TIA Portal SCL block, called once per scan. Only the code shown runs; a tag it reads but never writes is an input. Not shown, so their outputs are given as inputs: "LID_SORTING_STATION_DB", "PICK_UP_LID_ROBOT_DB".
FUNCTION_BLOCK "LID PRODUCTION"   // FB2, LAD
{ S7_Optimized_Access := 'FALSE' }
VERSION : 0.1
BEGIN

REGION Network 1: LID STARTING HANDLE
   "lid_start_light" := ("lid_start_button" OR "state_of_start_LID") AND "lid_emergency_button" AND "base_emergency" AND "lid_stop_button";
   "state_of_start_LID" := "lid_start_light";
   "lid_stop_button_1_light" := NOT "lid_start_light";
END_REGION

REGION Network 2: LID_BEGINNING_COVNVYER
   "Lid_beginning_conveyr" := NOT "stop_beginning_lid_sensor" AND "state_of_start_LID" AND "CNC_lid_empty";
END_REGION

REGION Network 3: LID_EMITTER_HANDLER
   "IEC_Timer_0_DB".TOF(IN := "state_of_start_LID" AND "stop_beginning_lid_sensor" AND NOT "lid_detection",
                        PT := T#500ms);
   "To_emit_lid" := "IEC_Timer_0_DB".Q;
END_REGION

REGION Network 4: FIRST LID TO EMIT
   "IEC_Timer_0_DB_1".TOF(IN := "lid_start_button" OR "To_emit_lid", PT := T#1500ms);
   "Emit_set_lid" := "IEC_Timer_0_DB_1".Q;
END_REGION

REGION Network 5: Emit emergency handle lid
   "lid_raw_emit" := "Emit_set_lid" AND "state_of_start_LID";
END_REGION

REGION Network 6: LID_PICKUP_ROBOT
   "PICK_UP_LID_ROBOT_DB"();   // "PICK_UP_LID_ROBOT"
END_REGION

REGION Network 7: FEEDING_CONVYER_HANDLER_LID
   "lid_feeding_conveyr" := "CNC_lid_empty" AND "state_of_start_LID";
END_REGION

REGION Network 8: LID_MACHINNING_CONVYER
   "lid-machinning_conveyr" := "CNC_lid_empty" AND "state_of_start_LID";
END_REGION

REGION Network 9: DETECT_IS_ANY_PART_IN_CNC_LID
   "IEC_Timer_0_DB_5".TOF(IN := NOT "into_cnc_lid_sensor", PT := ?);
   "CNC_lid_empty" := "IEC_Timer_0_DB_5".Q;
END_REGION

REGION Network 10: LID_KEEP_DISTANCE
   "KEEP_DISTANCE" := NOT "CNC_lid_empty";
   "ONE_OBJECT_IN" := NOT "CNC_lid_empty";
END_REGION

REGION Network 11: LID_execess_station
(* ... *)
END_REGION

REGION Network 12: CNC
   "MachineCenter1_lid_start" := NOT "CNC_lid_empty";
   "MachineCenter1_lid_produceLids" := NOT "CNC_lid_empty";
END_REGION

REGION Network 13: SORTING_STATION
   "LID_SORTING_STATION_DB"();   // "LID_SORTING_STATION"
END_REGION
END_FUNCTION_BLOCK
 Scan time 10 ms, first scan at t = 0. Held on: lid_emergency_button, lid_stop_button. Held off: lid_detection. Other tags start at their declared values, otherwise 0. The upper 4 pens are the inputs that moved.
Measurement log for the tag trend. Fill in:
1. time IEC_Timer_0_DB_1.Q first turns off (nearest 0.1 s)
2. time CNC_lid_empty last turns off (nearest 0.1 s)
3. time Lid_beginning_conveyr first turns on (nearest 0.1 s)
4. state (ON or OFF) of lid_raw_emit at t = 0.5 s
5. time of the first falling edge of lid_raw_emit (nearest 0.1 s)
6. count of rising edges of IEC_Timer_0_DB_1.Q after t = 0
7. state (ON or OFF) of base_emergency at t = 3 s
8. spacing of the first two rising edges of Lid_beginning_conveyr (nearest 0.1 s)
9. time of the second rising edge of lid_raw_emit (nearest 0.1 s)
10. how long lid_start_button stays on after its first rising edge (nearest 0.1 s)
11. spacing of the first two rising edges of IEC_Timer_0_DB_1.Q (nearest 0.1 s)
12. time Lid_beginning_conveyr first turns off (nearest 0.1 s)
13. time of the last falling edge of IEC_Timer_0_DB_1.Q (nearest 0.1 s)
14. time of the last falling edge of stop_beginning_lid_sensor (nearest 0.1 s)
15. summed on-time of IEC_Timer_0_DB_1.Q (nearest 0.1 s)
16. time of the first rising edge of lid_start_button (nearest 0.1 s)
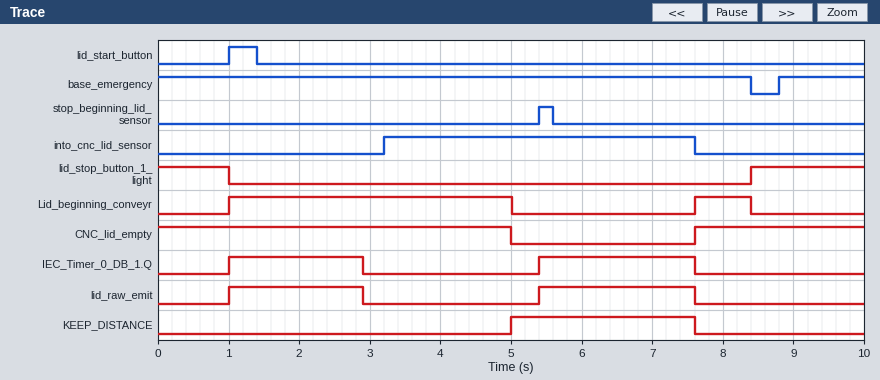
2.9 s
5.0 s
1.0 s
OFF
2.9 s
2
ON
6.6 s
5.4 s
0.4 s
4.4 s
5.0 s
7.6 s
5.6 s
4.1 s
1.0 s
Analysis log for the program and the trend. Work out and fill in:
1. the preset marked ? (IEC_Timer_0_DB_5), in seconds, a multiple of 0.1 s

1.8 s
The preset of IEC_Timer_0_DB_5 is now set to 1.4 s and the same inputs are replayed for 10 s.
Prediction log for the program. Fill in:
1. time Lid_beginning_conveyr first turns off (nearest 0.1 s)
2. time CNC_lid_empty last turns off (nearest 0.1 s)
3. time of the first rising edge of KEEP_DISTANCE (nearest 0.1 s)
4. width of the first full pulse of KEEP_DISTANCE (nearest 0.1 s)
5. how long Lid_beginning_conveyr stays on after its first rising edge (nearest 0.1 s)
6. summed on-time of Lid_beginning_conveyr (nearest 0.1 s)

4.6 s
4.6 s
4.6 s
3.0 s
3.6 s
4.4 s
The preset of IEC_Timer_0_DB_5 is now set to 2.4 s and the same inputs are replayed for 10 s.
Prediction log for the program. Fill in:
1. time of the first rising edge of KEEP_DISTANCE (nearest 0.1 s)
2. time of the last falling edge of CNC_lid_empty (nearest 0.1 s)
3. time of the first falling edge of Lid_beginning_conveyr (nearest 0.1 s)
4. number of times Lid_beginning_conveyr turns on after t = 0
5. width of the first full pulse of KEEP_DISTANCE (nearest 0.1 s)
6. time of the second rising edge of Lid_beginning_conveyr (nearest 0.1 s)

5.6 s
5.6 s
5.4 s
3
2.0 s
5.6 s
